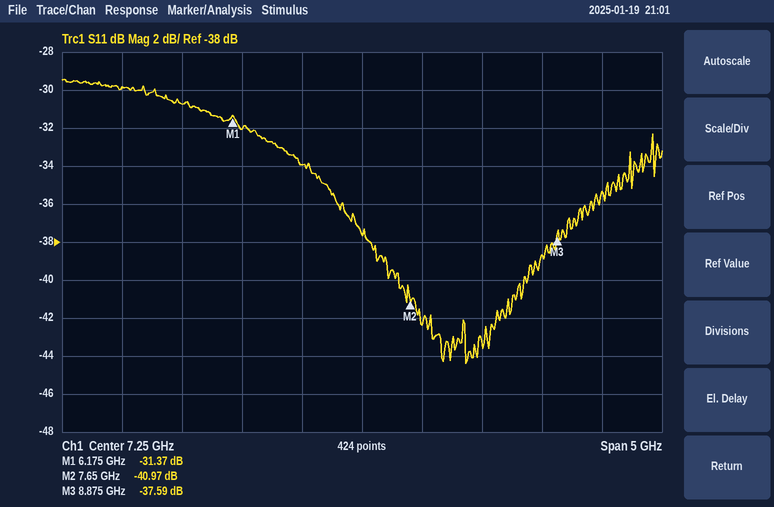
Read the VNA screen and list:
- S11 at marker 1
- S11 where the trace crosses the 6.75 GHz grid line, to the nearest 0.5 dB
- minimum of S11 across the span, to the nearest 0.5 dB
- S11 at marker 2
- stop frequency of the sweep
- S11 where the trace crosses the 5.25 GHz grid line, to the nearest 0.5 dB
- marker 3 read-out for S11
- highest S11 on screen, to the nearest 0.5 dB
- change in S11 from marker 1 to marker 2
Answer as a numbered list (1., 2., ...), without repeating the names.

1. -31.37 dB
2. -34.0 dB
3. -44.5 dB
4. -40.97 dB
5. 9.75 GHz
6. -30.0 dB
7. -37.59 dB
8. -29.5 dB
9. -9.60 dB
